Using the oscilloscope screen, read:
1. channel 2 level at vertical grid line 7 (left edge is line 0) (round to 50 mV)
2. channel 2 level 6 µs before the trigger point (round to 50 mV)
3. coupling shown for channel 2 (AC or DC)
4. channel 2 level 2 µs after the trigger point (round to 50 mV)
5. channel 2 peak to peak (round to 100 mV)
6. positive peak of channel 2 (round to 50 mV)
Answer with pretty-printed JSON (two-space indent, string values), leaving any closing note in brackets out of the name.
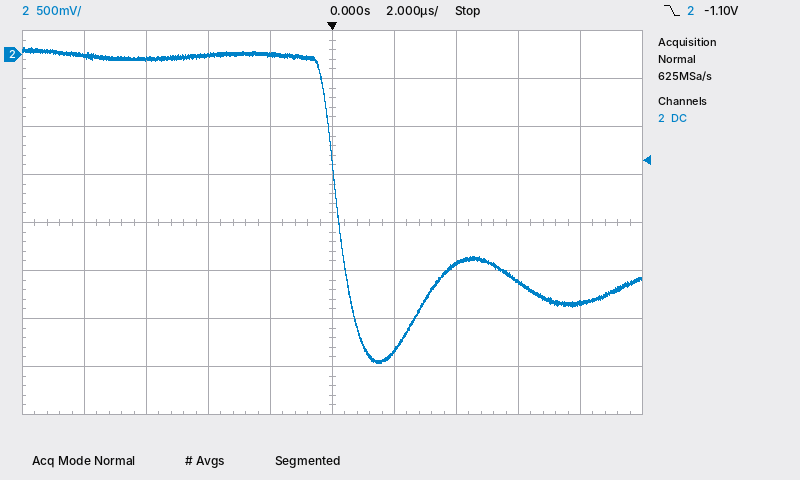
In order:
{
  "channel 2 level at vertical grid line 7 (left edge is line 0)": "-2.20 V",
  "channel 2 level 6 µs before the trigger point": "-50 mV",
  "coupling shown for channel 2": "DC",
  "channel 2 level 2 µs after the trigger point": "-3.10 V",
  "channel 2 peak to peak": "3.30 V",
  "positive peak of channel 2": "50 mV"
}
